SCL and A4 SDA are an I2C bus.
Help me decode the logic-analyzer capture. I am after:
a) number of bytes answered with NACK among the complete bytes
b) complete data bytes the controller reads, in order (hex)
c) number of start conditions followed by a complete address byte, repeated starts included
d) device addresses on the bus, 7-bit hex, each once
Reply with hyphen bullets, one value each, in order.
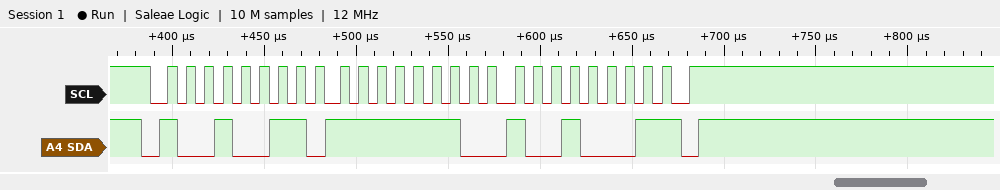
- 1
- FE 91
- 1
- 0x49
